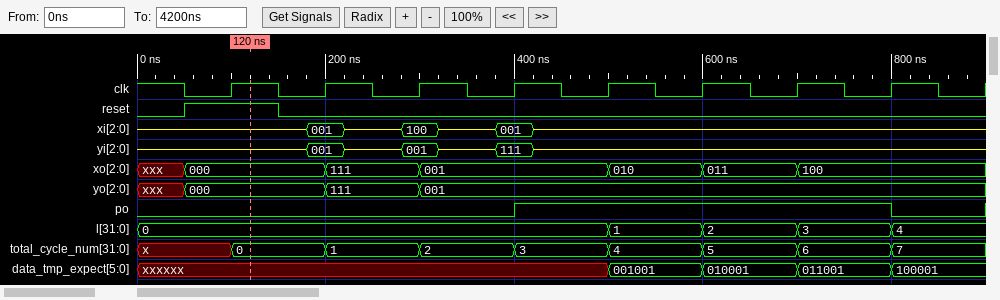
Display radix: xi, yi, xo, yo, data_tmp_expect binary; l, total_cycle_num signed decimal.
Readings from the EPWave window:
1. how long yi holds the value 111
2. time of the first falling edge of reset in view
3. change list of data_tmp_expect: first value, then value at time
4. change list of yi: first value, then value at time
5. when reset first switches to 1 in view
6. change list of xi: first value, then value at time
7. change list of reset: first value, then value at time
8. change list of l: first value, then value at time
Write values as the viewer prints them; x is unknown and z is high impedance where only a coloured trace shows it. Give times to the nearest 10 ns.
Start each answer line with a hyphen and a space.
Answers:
- 40 ns
- 150 ns
- xxxxxx, 001001 at 500 ns, 010001 at 600 ns, 011001 at 700 ns, 100001 at 800 ns
- z, 001 at 180 ns, z at 220 ns, 001 at 280 ns, z at 320 ns, 111 at 380 ns, z at 420 ns
- 50 ns
- z, 001 at 180 ns, z at 220 ns, 100 at 280 ns, z at 320 ns, 001 at 380 ns, z at 420 ns
- 0, 1 at 50 ns, 0 at 150 ns
- 0, 1 at 500 ns, 2 at 600 ns, 3 at 700 ns, 4 at 800 ns
